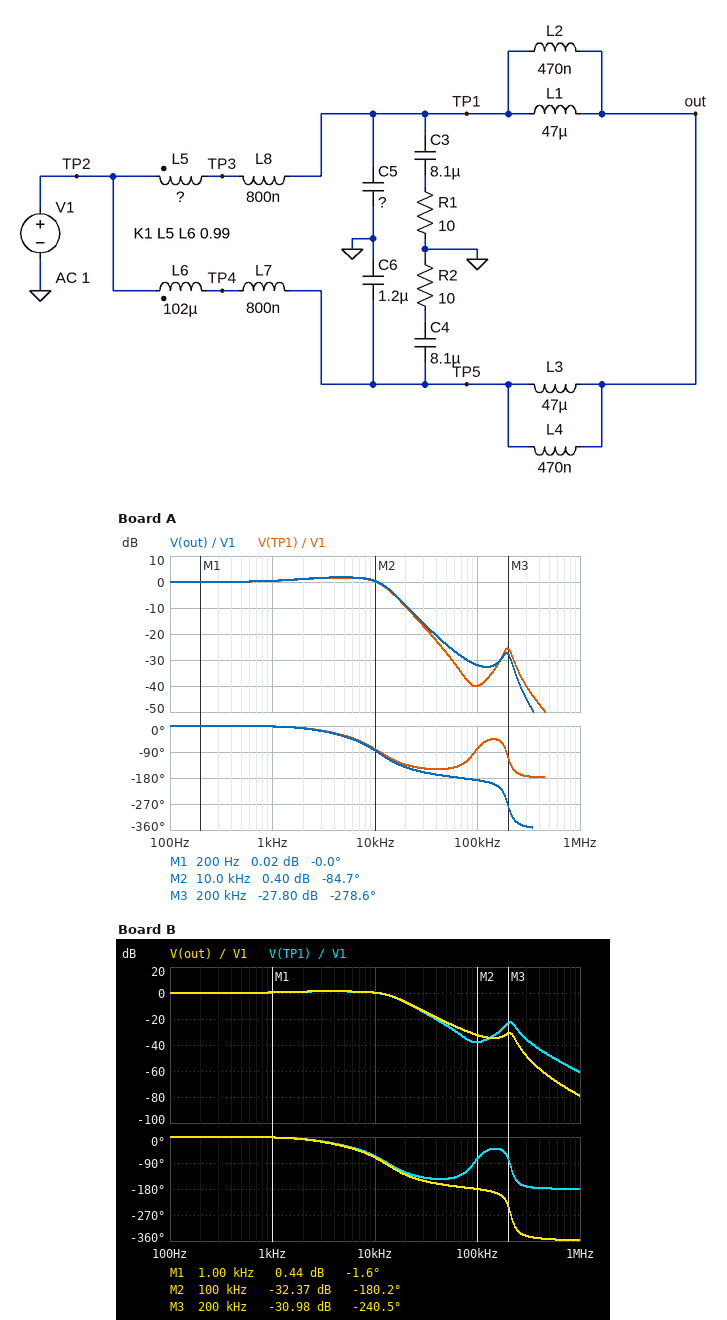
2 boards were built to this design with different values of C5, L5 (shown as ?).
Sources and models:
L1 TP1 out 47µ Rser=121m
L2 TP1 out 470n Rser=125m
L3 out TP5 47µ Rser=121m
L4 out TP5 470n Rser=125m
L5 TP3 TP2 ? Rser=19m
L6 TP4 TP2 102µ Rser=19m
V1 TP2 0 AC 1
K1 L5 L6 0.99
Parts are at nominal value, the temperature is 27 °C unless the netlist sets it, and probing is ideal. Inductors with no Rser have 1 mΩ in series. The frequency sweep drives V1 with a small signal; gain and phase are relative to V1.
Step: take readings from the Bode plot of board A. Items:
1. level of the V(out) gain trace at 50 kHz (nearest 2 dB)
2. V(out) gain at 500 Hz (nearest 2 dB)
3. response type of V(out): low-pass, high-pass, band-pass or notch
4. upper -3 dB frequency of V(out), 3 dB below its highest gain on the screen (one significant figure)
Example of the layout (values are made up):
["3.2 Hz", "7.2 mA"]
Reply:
["-24 dB", "0 dB", "low-pass", "10 kHz"]
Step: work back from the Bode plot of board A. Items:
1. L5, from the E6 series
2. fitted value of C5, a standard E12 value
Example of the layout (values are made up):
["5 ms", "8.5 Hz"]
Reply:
["68 µH", "3.3 µF"]
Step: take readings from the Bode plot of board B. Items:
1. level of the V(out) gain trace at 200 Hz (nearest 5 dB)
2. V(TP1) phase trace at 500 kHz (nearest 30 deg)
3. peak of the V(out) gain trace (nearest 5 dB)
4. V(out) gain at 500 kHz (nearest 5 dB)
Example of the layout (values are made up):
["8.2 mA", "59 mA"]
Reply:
["0 dB", "-180 deg", "0 dB", "-65 dB"]
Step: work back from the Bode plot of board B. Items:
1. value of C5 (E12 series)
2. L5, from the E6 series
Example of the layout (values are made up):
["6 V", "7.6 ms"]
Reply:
["2.2 µF", "68 µH"]
